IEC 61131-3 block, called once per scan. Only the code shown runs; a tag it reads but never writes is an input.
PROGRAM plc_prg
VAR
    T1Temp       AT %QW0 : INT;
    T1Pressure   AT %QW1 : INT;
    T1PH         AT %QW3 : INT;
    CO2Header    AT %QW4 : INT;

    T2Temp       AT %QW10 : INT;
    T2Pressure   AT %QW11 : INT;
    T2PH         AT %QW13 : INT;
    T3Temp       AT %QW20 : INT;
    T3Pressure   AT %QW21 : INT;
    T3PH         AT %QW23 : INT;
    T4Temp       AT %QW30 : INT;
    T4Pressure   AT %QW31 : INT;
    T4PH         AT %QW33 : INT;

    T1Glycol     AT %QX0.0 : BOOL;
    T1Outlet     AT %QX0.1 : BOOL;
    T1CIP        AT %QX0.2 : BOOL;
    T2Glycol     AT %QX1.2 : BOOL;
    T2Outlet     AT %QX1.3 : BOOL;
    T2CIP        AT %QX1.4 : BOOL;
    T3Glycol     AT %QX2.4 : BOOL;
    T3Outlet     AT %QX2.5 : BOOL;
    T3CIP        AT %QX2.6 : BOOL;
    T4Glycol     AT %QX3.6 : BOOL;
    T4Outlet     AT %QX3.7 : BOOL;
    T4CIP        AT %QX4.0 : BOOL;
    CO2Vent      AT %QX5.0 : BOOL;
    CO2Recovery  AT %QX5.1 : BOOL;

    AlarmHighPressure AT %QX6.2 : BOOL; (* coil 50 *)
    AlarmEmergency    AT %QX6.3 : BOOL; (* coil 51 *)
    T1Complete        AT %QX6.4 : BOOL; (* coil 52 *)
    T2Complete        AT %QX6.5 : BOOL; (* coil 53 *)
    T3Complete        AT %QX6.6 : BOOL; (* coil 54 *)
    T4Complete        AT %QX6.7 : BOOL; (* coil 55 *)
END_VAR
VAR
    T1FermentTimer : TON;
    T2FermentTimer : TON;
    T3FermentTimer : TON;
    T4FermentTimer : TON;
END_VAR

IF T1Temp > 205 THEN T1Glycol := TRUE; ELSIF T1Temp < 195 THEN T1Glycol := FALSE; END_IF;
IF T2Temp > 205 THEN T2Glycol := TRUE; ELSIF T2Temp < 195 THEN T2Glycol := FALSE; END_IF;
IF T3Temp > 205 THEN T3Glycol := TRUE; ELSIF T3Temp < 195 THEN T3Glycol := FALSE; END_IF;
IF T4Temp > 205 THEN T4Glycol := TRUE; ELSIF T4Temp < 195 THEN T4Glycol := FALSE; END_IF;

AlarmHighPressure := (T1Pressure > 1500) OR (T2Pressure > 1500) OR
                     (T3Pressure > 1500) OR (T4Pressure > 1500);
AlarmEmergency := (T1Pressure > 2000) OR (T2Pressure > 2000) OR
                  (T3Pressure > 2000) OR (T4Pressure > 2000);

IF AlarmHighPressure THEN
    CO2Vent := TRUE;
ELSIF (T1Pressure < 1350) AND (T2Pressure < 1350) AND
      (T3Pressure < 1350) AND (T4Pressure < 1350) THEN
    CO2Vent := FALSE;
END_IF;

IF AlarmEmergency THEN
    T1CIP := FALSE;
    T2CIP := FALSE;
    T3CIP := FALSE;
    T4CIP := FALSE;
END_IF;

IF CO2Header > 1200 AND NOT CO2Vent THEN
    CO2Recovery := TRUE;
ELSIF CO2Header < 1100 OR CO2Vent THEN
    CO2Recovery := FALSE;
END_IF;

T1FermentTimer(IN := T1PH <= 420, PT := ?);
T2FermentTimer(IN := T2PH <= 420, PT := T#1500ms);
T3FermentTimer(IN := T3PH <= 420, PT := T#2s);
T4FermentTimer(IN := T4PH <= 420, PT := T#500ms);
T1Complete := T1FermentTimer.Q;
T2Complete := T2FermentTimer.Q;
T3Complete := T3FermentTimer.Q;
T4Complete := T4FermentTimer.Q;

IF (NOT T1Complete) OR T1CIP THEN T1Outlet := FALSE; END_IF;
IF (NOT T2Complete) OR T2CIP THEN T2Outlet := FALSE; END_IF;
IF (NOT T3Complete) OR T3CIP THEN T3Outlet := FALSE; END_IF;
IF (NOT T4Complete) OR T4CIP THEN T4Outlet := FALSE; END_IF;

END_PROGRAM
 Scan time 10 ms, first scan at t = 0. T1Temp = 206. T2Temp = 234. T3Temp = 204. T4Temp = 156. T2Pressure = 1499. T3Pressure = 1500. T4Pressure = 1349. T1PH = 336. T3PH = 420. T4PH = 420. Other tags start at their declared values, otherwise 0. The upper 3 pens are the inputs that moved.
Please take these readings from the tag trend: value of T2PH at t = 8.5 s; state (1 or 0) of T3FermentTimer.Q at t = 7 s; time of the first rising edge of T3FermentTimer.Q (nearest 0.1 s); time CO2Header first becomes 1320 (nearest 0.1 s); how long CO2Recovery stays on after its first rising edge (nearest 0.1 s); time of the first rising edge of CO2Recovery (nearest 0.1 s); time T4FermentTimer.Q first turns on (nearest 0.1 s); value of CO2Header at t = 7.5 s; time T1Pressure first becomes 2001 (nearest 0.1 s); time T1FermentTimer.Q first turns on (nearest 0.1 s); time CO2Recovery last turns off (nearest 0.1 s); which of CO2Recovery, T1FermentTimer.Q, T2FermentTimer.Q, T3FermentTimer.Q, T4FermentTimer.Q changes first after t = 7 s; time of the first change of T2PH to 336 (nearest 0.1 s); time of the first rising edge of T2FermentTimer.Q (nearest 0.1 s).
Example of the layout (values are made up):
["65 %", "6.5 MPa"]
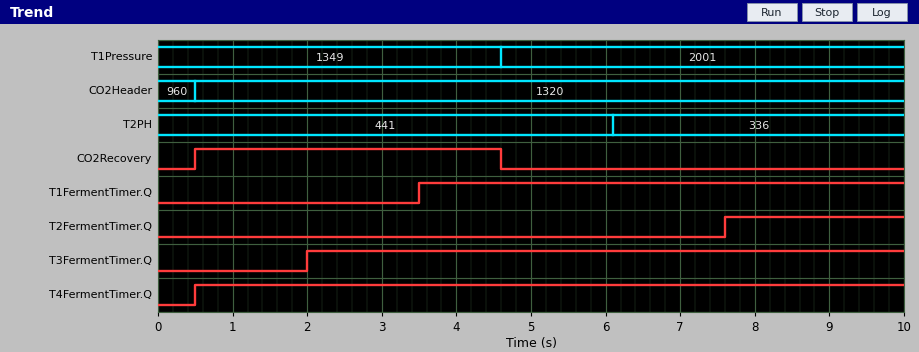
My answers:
["336", "1", "2.0 s", "0.5 s", "4.1 s", "0.5 s", "0.5 s", "1320", "4.6 s", "3.5 s", "4.6 s", "T2FermentTimer.Q", "6.1 s", "7.6 s"]
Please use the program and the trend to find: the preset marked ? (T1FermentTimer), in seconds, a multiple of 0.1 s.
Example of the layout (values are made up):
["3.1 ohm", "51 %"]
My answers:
["3.5 s"]
